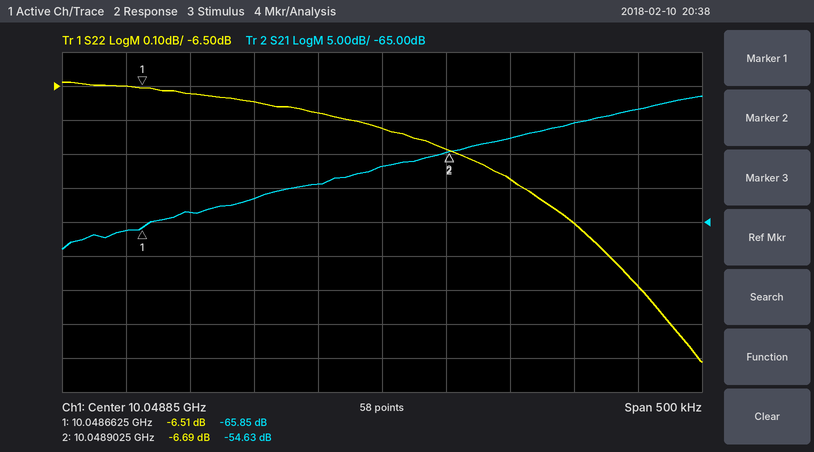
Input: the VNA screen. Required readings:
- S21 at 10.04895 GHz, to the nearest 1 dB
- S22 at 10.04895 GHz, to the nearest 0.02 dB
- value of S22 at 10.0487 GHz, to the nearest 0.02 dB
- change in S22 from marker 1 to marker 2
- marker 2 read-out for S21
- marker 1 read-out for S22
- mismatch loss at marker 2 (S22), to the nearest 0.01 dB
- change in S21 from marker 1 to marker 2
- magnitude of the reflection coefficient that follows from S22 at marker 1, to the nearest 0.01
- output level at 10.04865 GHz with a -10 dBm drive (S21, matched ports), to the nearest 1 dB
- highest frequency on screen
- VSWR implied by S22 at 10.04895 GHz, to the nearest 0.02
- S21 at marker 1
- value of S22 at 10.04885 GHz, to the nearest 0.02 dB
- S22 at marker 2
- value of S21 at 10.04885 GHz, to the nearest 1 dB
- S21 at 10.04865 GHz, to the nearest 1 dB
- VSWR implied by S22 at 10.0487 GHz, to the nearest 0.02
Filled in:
-53 dB
-6.78 dB
-6.52 dB
-0.18 dB
-54.63 dB
-6.51 dB
1.05 dB
11.22 dB
0.47
-76 dBm
10.0491 GHz
2.70
-65.85 dB
-6.62 dB
-6.69 dB
-57 dB
-66 dB
2.78
